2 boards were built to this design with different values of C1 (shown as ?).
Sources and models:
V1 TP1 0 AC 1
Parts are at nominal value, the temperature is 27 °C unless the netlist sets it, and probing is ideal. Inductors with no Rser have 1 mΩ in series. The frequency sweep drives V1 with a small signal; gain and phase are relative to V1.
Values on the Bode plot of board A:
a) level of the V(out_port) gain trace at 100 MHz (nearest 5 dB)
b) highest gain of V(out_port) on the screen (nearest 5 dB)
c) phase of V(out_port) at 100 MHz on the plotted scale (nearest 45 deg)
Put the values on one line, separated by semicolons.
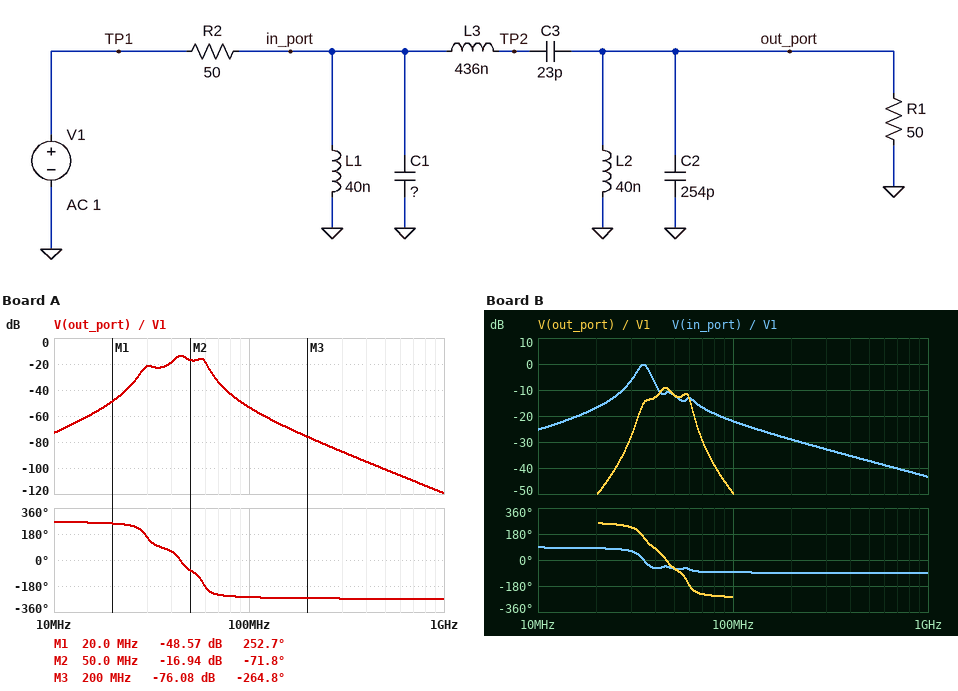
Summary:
-55 dB; -15 dB; -270 deg
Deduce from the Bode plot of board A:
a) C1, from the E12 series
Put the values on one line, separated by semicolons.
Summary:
680 pF
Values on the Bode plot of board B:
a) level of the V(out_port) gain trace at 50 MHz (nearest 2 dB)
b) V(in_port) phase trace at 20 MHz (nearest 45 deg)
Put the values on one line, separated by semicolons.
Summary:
-12 dB; 90 deg
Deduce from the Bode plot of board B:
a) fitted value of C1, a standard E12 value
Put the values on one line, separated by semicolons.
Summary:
470 pF
